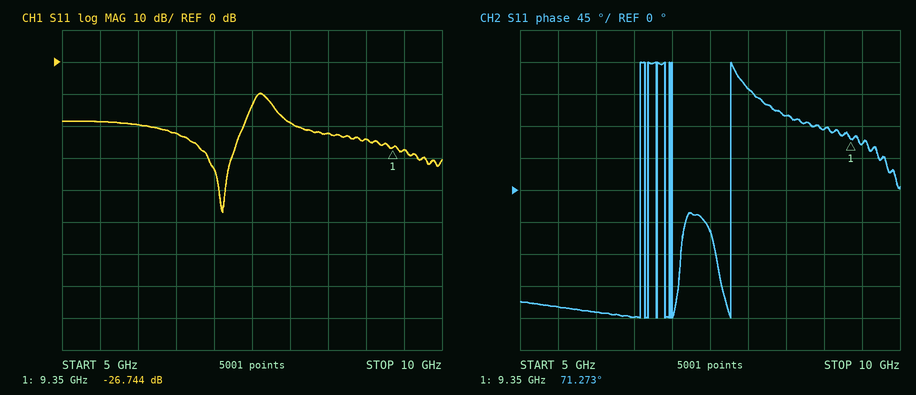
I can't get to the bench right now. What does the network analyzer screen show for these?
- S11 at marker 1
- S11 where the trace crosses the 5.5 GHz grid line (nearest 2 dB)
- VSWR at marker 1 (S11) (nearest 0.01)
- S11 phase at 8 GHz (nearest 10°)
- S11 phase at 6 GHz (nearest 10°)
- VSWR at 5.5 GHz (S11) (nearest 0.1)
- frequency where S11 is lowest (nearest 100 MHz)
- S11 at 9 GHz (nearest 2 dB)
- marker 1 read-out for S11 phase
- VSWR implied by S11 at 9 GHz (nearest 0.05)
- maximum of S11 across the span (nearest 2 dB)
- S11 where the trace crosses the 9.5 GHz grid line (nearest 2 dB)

-26.744 dB
-18 dB
1.10
140°
-170°
1.3
7.1 GHz
-24 dB
71.273°
1.15
-10 dB
-28 dB
